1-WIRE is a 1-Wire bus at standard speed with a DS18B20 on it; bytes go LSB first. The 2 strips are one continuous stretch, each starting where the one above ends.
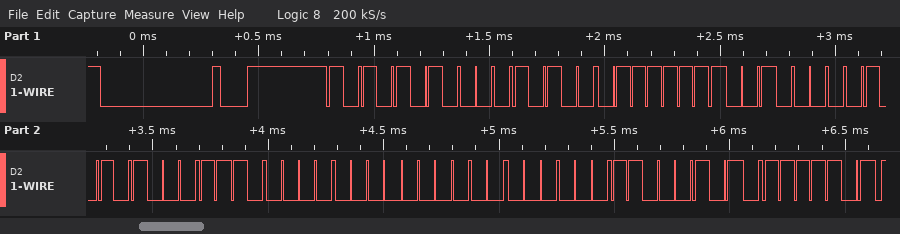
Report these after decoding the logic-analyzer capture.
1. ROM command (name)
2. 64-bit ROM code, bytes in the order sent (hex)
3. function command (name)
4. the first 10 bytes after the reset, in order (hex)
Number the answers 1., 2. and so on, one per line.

1. Match ROM
2. 28 FE 04 15 07 00 00 A3
3. Read Scratchpad
4. 55 28 FE 04 15 07 00 00 A3 BE
